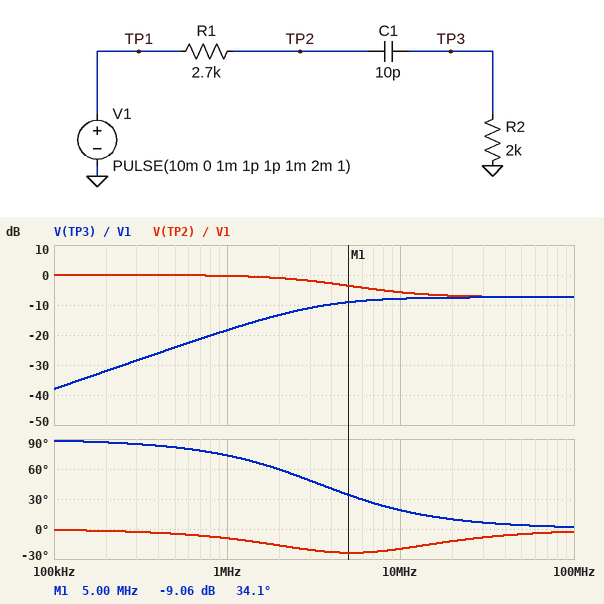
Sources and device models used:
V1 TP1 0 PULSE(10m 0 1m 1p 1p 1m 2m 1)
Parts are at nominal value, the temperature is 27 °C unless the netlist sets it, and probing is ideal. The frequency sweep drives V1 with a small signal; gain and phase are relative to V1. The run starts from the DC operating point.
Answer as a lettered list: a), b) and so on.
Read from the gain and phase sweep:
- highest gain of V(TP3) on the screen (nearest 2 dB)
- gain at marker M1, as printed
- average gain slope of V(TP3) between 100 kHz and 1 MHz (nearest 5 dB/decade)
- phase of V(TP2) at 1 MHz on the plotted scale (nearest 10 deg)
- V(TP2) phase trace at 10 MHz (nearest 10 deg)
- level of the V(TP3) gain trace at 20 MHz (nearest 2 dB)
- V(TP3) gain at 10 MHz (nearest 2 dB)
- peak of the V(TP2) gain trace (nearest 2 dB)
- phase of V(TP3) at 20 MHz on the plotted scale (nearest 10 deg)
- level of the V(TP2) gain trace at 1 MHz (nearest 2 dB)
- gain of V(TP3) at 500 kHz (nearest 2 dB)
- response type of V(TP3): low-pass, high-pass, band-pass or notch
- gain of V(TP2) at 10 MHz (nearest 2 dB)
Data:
a) -8 dB
b) -9.06 dB
c) 20 dB/decade
d) -10 deg
e) -20 deg
f) -8 dB
g) -8 dB
h) 0 dB
i) 10 deg
j) 0 dB
k) -24 dB
l) high-pass
m) -6 dB
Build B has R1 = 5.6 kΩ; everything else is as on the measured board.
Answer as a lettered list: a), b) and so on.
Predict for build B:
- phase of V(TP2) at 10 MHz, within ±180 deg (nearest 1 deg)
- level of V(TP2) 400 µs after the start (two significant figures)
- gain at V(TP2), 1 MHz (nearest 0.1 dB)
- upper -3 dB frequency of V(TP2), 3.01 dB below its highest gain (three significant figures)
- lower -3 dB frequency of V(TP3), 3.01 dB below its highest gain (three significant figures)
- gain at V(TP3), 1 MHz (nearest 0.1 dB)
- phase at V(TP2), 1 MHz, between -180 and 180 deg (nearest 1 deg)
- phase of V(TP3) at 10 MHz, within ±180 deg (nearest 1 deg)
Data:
a) -27 deg
b) 10 mV
c) -0.8 dB
d) 2.26 MHz
e) 2.09 MHz
f) -18.9 dB
g) -18 deg
h) 12 deg
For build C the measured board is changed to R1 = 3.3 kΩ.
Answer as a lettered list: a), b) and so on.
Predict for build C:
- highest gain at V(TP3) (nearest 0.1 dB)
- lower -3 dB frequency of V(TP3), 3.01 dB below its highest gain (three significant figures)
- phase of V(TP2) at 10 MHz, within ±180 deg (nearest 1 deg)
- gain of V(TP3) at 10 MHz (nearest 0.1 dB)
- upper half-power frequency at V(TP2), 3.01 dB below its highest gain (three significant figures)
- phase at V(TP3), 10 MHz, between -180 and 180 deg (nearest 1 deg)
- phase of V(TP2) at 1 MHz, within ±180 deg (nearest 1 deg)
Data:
a) -8.5 dB
b) 3.00 MHz
c) -22 deg
d) -8.8 dB
e) 3.55 MHz
f) 17 deg
g) -11 deg
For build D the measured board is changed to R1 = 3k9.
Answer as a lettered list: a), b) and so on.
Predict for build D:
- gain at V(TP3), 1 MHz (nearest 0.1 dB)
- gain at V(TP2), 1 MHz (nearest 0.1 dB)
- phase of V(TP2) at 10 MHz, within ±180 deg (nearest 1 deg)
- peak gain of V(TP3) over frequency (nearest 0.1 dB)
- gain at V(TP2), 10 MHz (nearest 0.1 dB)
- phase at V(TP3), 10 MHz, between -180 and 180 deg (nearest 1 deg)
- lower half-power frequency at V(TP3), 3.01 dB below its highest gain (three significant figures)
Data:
a) -18.6 dB
b) -0.5 dB
c) -23 deg
d) -9.4 dB
e) -7.6 dB
f) 15 deg
g) 2.70 MHz
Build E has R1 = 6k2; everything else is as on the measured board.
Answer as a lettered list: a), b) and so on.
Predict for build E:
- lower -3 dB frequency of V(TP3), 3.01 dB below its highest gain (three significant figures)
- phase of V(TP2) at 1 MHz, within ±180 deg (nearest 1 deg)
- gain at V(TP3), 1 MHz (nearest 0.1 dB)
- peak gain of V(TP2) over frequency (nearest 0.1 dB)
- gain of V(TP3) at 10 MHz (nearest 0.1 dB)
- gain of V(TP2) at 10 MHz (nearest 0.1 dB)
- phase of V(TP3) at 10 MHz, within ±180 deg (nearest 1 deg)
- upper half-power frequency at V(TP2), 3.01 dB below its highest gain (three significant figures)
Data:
a) 1.94 MHz
b) -20 deg
c) -19.0 dB
d) 0 dB
e) -12.4 dB
f) -10.3 dB
g) 11 deg
h) 2.07 MHz
